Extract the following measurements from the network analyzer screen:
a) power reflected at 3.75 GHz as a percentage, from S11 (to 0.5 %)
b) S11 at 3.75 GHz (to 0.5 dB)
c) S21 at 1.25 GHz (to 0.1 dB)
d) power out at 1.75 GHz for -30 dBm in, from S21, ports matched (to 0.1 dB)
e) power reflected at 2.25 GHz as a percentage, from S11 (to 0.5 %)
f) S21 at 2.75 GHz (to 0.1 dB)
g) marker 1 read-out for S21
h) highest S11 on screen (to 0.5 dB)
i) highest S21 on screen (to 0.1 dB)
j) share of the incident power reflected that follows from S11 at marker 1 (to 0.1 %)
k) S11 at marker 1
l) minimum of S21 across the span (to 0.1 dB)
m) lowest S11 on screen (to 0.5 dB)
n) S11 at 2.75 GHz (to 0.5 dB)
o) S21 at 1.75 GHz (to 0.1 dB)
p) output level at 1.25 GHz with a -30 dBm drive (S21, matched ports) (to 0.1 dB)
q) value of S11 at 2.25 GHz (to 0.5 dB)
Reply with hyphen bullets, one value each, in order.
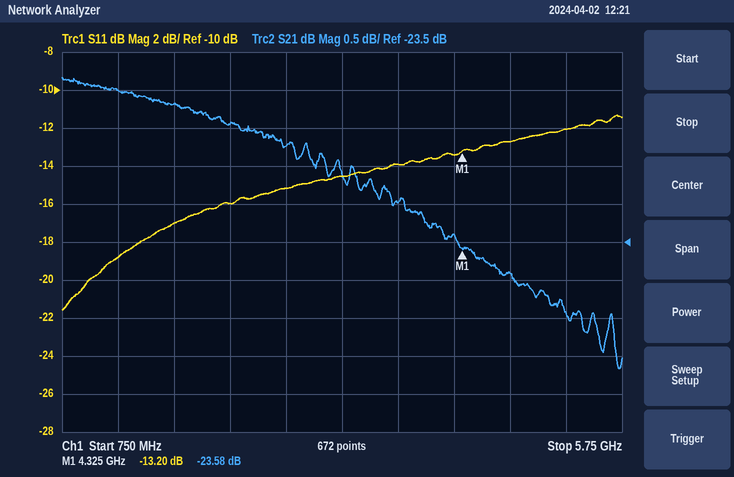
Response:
- 4.0 %
- -14.0 dB
- -21.5 dB
- -51.7 dBm
- 2.5 %
- -22.2 dB
- -23.58 dB
- -11.5 dB
- -21.3 dB
- 4.8 %
- -13.20 dB
- -25.2 dB
- -21.5 dB
- -15.0 dB
- -21.7 dB
- -51.5 dBm
- -16.0 dB
